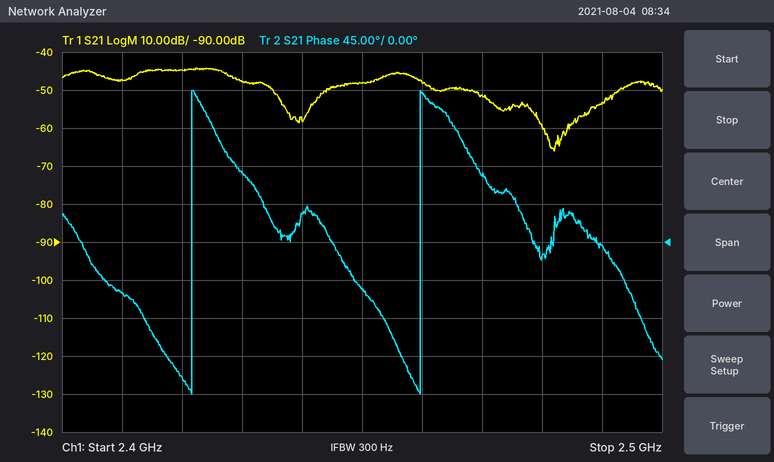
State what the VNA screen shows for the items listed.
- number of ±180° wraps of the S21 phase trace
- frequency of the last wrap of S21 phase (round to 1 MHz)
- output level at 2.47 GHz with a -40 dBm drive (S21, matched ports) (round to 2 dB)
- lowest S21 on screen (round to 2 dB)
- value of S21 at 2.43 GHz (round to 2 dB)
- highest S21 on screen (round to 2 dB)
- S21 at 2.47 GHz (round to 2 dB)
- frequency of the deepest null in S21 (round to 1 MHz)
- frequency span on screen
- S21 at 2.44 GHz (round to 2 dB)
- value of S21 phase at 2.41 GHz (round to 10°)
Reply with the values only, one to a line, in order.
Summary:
2
2.460 GHz
-92 dBm
-66 dB
-48 dB
-44 dB
-52 dB
2.482 GHz
100 MHz
-58 dB
-60°
